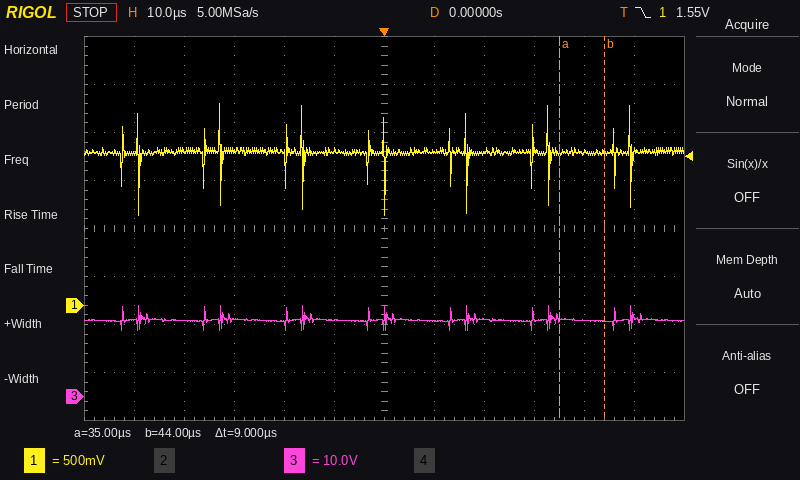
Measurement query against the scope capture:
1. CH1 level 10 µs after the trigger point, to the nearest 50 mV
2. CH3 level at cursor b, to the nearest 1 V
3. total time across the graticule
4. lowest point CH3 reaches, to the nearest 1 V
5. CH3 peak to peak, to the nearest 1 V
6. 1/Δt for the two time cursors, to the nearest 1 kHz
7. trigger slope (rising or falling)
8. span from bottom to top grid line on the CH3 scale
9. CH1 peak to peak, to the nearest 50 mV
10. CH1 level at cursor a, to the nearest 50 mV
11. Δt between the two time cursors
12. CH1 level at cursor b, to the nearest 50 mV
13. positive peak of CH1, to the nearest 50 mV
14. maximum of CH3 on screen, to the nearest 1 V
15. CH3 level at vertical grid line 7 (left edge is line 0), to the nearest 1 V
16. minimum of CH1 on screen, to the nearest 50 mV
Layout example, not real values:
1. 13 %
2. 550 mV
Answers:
1. 1.60 V
2. 16 V
3. 120 µs
4. 14 V
5. 5 V
6. 111 kHz
7. falling
8. 80 V
9. 1.15 V
10. 1.60 V
11. 9 µs
12. 1.60 V
13. 2.10 V
14. 19 V
15. 16 V
16. 950 mV
